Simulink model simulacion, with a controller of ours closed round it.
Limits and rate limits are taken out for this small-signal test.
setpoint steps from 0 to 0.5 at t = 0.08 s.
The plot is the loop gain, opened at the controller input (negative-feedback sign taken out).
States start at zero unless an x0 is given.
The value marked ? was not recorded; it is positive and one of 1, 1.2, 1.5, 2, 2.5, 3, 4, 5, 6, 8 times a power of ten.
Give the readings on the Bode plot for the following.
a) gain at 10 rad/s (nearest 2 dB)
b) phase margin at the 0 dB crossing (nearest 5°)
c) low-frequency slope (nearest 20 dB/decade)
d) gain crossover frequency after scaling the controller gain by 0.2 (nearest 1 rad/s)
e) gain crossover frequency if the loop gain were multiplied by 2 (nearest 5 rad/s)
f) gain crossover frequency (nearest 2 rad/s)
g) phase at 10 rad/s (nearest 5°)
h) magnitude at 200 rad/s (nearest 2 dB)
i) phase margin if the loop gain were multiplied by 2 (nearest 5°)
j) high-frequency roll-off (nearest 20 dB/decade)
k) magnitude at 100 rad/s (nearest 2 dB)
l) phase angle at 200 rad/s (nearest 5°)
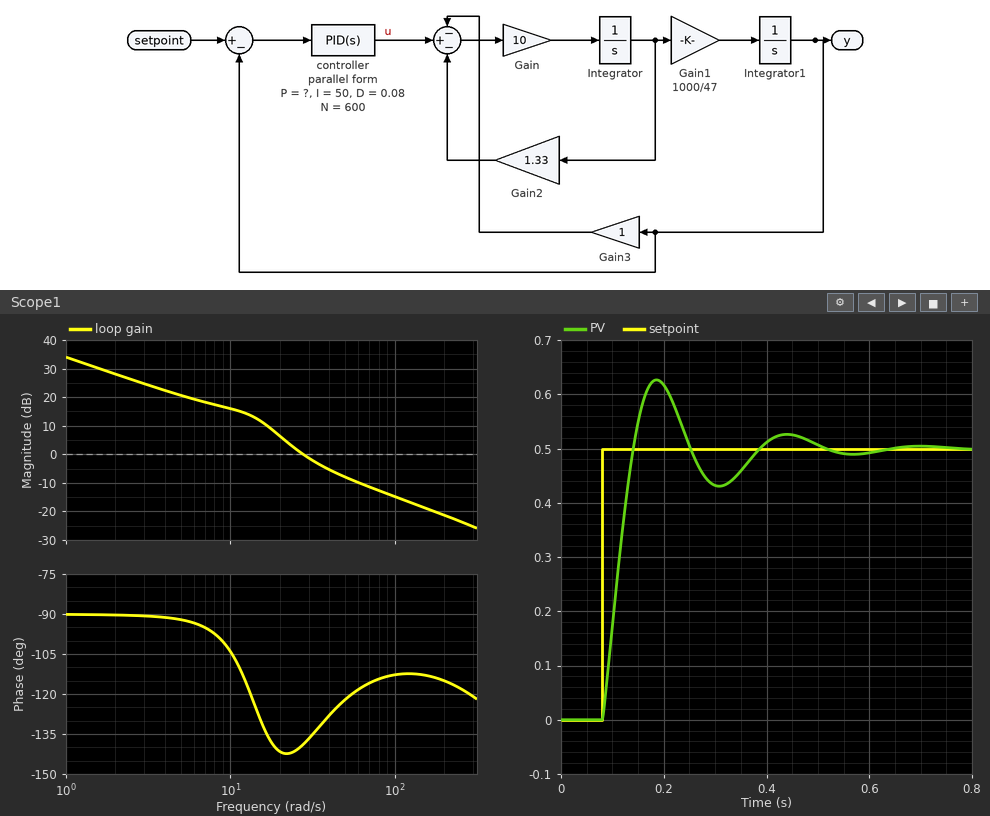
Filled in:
16 dB
40°
-20 dB/decade
13 rad/s
40 rad/s
28 rad/s
-105°
-22 dB
55°
-20 dB/decade
-14 dB
-115°
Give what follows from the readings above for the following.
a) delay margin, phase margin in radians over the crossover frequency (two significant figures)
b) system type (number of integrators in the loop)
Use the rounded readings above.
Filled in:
0.025 s
1
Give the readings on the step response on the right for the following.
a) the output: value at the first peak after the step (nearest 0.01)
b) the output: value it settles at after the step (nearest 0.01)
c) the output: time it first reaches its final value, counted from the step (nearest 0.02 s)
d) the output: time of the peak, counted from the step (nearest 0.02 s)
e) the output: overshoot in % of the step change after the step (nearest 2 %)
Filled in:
0.63
0.50
0.06 s
0.10 s
26 %
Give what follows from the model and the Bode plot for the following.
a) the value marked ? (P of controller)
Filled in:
3
